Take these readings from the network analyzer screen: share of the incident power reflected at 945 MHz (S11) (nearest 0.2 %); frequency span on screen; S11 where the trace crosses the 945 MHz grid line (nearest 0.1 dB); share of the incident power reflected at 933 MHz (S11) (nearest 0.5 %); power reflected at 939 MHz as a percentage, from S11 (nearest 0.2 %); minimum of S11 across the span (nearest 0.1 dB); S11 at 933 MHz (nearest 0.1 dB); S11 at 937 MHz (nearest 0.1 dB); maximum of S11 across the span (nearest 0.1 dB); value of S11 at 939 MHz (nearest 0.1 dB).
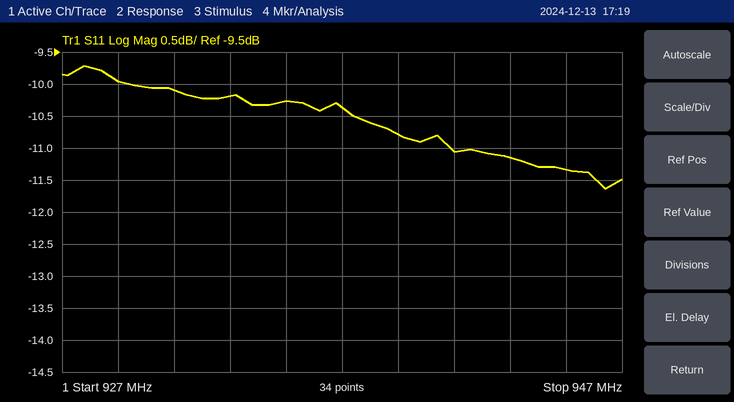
7.4 %
20 MHz
-11.3 dB
9.5 %
8.4 %
-11.6 dB
-10.2 dB
-10.4 dB
-9.7 dB
-10.8 dB
